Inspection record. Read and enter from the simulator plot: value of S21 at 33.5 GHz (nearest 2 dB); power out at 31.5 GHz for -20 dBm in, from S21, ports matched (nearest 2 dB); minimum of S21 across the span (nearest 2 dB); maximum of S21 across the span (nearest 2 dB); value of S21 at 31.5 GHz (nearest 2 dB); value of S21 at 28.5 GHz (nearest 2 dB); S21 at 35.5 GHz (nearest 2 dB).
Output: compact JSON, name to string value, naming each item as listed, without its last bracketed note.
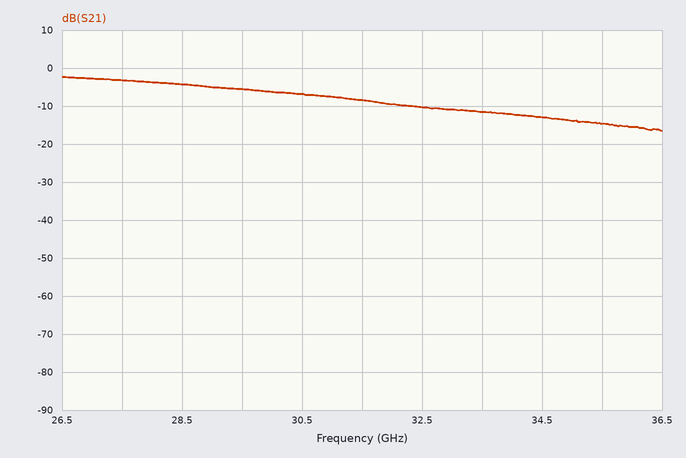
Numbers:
{"value of S21 at 33.5 GHz": "-12 dB", "power out at 31.5 GHz for -20 dBm in, from S21, ports matched": "-28 dBm", "minimum of S21 across the span": "-16 dB", "maximum of S21 across the span": "-2 dB", "value of S21 at 31.5 GHz": "-8 dB", "value of S21 at 28.5 GHz": "-4 dB", "S21 at 35.5 GHz": "-14 dB"}
